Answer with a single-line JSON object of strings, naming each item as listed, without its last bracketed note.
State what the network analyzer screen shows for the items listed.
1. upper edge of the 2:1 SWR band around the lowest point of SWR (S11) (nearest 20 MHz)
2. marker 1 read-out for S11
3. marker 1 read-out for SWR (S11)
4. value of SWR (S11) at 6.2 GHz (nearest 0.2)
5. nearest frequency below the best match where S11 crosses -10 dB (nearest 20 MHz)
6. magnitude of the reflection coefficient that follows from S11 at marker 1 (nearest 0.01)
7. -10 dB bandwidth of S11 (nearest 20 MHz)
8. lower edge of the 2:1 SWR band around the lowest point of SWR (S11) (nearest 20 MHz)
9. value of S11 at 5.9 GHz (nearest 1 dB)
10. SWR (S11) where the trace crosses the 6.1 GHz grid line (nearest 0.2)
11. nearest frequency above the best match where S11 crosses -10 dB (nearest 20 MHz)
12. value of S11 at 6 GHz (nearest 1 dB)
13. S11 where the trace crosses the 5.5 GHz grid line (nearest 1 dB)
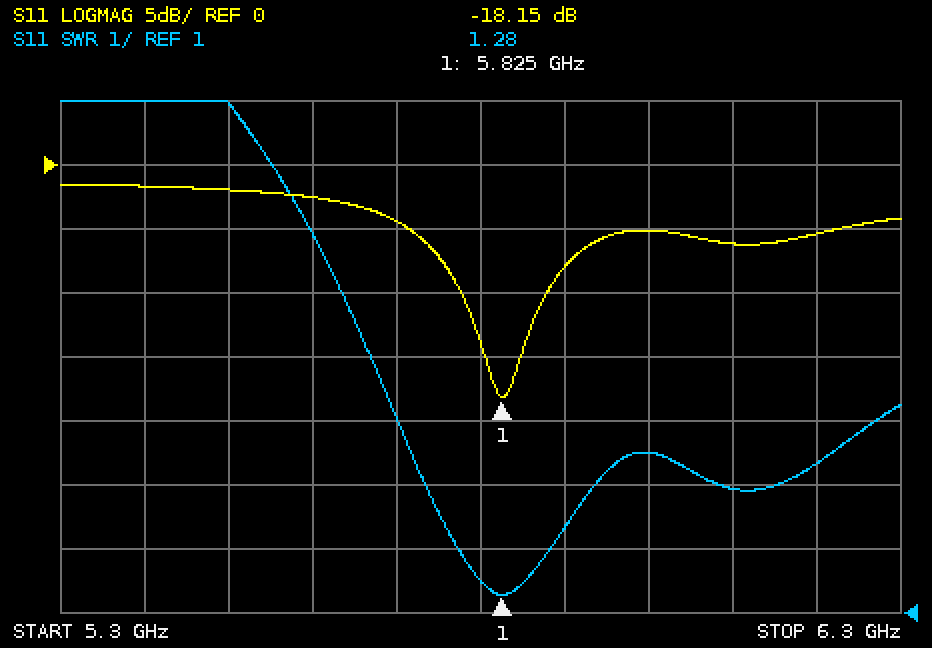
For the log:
{"upper edge of the 2:1 SWR band around the lowest point of SWR (S11)": "5.88 GHz", "marker 1 read-out for S11": "-18.15 dB", "marker 1 read-out for SWR": "1.28", "value of SWR (S11) at 6.2 GHz": "3.4", "nearest frequency below the best match where S11 crosses -10 dB": "5.78 GHz", "magnitude of the reflection coefficient that follows from S11 at marker 1": "0.12", "-10 dB bandwidth of S11": "100 MHz", "lower edge of the 2:1 SWR band around the lowest point of SWR (S11)": "5.78 GHz", "value of S11 at 5.9 GHz": "-8 dB", "SWR (S11) where the trace crosses the 6.1 GHz grid line": "3.0", "nearest frequency above the best match where S11 crosses -10 dB": "5.88 GHz", "value of S11 at 6 GHz": "-5 dB", "S11 where the trace crosses the 5.5 GHz grid line": "-2 dB"}
